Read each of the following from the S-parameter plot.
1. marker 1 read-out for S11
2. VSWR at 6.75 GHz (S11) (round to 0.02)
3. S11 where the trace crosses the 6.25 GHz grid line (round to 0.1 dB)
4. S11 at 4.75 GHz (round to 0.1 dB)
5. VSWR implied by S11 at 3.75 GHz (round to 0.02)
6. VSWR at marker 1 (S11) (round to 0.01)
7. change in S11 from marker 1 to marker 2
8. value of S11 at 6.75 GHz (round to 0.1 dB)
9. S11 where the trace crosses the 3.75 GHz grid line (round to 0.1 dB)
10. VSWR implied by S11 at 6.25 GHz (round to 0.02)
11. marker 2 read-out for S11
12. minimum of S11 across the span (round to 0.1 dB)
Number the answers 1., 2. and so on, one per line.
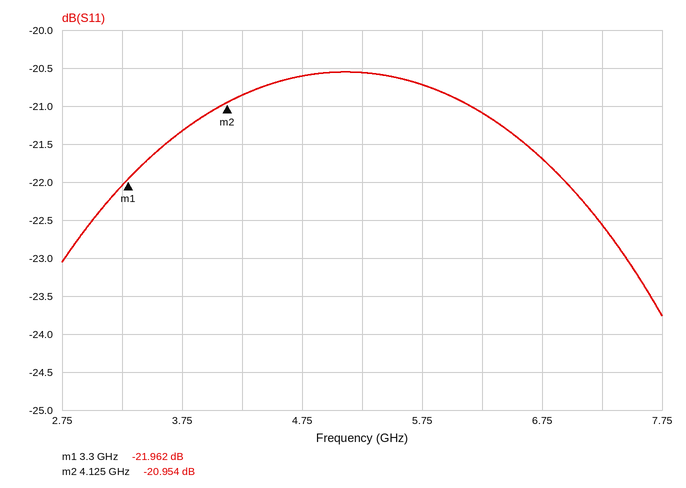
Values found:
1. -21.962 dB
2. 1.18
3. -21.1 dB
4. -20.6 dB
5. 1.18
6. 1.17
7. 1.008 dB
8. -21.7 dB
9. -21.3 dB
10. 1.20
11. -20.954 dB
12. -23.8 dB
